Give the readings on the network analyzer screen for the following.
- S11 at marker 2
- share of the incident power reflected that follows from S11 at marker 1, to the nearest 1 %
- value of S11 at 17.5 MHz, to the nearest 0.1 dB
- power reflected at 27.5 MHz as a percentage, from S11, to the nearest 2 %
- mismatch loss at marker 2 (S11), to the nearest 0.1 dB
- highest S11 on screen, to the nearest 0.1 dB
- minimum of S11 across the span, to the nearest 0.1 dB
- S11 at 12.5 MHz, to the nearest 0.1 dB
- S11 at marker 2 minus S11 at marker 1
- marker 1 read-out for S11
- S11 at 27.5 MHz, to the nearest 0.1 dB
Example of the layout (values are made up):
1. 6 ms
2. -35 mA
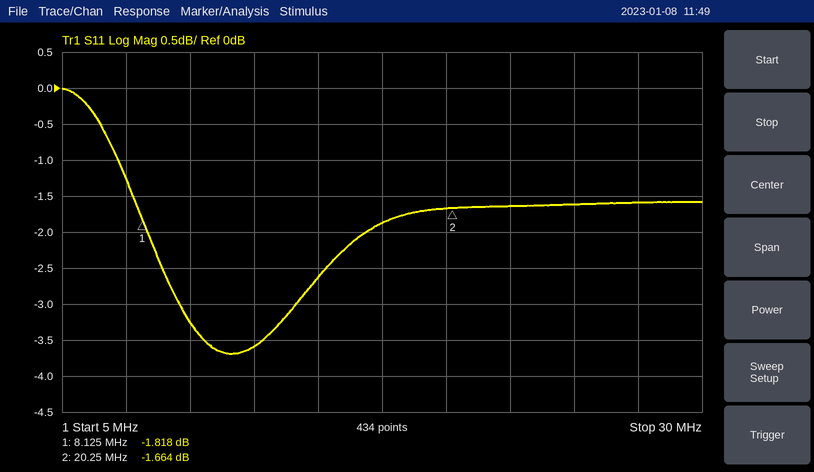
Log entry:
1. -1.664 dB
2. 66 %
3. -1.9 dB
4. 70 %
5. 5.0 dB
6. 0.0 dB
7. -3.7 dB
8. -3.6 dB
9. 0.154 dB
10. -1.818 dB
11. -1.6 dB
